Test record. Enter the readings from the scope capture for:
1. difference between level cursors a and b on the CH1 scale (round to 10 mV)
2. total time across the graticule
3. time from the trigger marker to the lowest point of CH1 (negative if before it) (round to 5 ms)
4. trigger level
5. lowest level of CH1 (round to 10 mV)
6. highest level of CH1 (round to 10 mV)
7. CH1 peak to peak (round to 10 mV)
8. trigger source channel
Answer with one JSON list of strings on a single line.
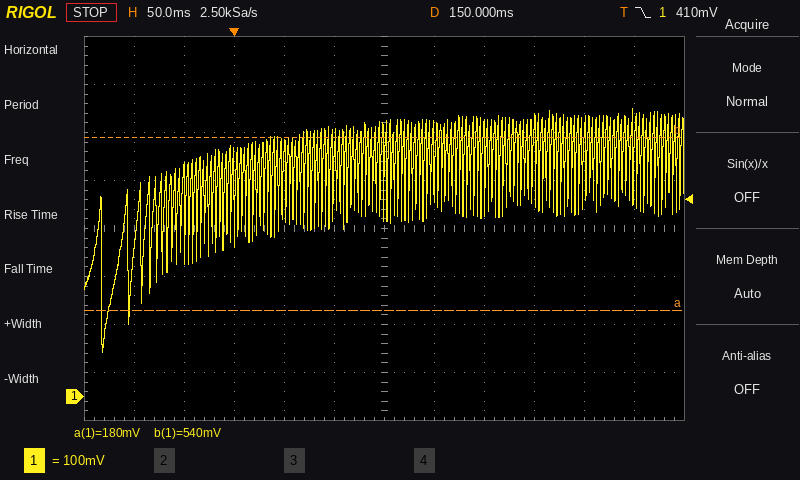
["360 mV", "600 ms", "-130 ms", "410 mV", "90 mV", "600 mV", "510 mV", "CH1"]
